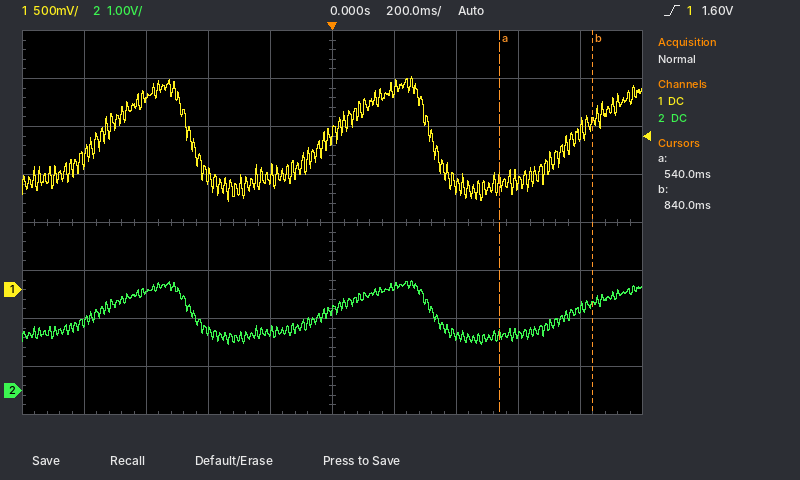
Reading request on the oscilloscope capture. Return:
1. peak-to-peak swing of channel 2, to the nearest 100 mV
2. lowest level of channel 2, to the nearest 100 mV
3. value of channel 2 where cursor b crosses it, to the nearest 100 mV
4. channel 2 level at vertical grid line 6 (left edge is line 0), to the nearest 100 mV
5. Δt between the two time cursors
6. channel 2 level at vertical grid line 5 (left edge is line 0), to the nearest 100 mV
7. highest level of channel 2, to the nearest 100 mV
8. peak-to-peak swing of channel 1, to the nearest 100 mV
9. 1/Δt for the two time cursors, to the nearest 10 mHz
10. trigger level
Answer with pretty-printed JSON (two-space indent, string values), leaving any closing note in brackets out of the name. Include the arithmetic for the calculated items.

{
  "peak-to-peak swing of channel 2, to the nearest 100 mV": "2.3 V − (1.0 V) = 1.3 V",
  "lowest level of channel 2, to the nearest 100 mV": "1.0 V",
  "value of channel 2 where cursor b crosses it, to the nearest 100 mV": "1.8 V",
  "channel 2 level at vertical grid line 6 (left edge is line 0), to the nearest 100 mV": "2.2 V",
  "Δt between the two time cursors": "840 ms − (540 ms) = 300 ms",
  "channel 2 level at vertical grid line 5 (left edge is line 0), to the nearest 100 mV": "1.7 V",
  "highest level of channel 2, to the nearest 100 mV": "2.3 V",
  "peak-to-peak swing of channel 1, to the nearest 100 mV": "1.30 V",
  "1/Δt for the two time cursors, to the nearest 10 mHz": "1 / 300 ms ≈ 3.33 Hz",
  "trigger level": "1.60 V"
}
